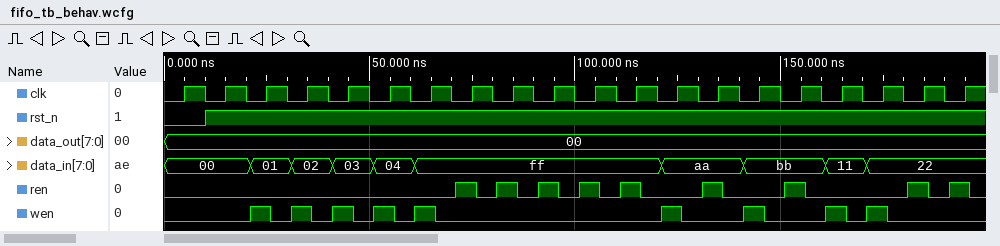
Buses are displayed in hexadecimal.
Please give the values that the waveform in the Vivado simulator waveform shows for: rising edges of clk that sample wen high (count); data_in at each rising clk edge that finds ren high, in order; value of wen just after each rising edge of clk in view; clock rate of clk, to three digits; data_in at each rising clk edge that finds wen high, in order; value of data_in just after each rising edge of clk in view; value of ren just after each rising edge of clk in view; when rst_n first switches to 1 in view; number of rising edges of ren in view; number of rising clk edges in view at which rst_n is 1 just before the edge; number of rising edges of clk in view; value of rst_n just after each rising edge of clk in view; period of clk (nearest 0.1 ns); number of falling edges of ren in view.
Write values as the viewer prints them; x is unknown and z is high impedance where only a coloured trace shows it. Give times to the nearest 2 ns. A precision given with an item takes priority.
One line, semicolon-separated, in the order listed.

9; ff, ff, ff, ff, ff, aa, bb, 22, 22; 0 0 1 1 1 1 1 0 0 0 0 0 1 0 1 0 1 1 0 0; 100 MHz; 01, 02, 03, 04, ff, aa, bb, 11, 22; 00, 00, 01, 02, 03, 04, ff, ff, ff, ff, ff, ff, aa, aa, bb, bb, 11, 22, 22, 22; 0 0 0 0 0 0 0 1 1 1 1 1 0 1 0 1 0 0 1 1; 10 ns; 9; 19; 20; 0 1 1 1 1 1 1 1 1 1 1 1 1 1 1 1 1 1 1 1; 10 ns; 9
